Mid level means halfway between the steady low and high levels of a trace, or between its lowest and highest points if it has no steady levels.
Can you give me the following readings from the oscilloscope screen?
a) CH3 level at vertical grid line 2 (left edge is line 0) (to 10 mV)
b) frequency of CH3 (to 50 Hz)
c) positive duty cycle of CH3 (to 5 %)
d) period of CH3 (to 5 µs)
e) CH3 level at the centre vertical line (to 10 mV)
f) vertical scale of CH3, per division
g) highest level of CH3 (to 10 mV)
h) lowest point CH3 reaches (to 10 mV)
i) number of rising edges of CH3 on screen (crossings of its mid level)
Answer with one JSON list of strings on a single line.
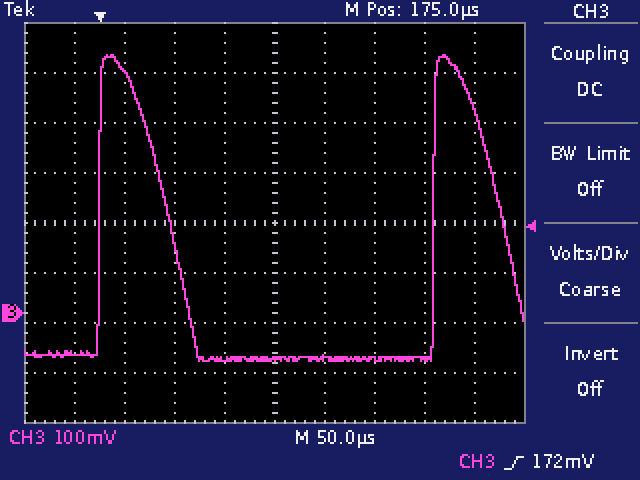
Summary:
["480 mV", "3.00 kHz", "20 %", "335 µs", "-90 mV", "100 mV", "520 mV", "-100 mV", "2"]
